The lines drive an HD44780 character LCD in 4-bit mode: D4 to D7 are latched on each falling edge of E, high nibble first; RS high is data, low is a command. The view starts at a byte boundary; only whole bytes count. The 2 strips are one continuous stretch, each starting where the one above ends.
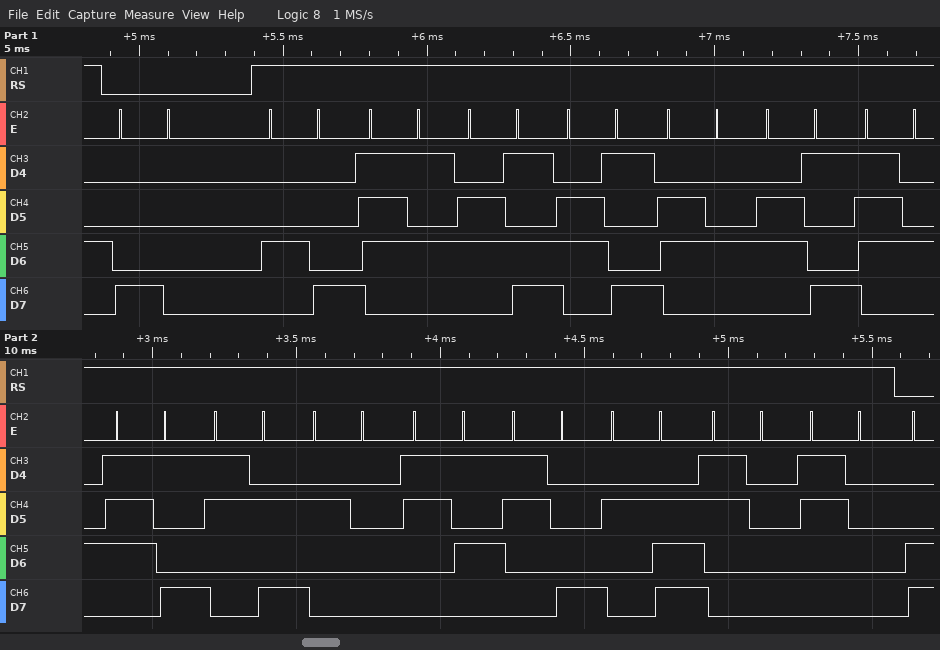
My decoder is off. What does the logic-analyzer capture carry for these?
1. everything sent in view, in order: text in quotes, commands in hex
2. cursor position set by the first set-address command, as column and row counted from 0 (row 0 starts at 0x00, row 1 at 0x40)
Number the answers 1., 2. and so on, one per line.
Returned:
1. 0x80 "Humidity: 58.00"
2. column 0, row 0
